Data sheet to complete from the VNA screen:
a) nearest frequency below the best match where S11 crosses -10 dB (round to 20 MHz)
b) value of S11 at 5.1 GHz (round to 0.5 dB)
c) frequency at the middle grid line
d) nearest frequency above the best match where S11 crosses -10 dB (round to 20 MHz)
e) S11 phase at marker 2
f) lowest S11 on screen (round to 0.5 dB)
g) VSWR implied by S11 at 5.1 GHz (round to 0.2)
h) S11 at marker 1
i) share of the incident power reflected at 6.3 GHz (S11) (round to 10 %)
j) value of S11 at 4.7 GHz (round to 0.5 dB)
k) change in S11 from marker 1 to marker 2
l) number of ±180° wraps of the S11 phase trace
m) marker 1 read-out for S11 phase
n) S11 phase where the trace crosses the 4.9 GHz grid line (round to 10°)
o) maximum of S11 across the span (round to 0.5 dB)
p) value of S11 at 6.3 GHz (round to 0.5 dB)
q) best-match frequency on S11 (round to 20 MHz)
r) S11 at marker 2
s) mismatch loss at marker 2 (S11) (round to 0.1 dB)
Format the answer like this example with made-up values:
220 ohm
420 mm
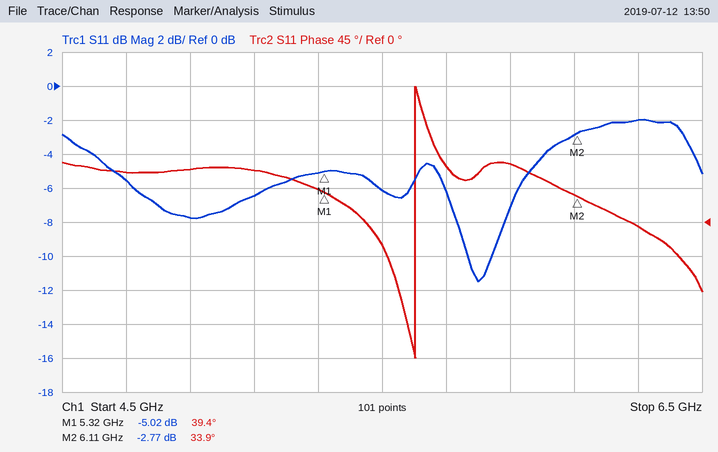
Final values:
5.76 GHz
-6.5 dB
5.5 GHz
5.84 GHz
33.9°
-11.5 dB
2.8
-5.02 dB
60 %
-5.5 dB
2.25 dB
1
39.4°
70°
-2.0 dB
-2.0 dB
5.80 GHz
-2.77 dB
3.3 dB
